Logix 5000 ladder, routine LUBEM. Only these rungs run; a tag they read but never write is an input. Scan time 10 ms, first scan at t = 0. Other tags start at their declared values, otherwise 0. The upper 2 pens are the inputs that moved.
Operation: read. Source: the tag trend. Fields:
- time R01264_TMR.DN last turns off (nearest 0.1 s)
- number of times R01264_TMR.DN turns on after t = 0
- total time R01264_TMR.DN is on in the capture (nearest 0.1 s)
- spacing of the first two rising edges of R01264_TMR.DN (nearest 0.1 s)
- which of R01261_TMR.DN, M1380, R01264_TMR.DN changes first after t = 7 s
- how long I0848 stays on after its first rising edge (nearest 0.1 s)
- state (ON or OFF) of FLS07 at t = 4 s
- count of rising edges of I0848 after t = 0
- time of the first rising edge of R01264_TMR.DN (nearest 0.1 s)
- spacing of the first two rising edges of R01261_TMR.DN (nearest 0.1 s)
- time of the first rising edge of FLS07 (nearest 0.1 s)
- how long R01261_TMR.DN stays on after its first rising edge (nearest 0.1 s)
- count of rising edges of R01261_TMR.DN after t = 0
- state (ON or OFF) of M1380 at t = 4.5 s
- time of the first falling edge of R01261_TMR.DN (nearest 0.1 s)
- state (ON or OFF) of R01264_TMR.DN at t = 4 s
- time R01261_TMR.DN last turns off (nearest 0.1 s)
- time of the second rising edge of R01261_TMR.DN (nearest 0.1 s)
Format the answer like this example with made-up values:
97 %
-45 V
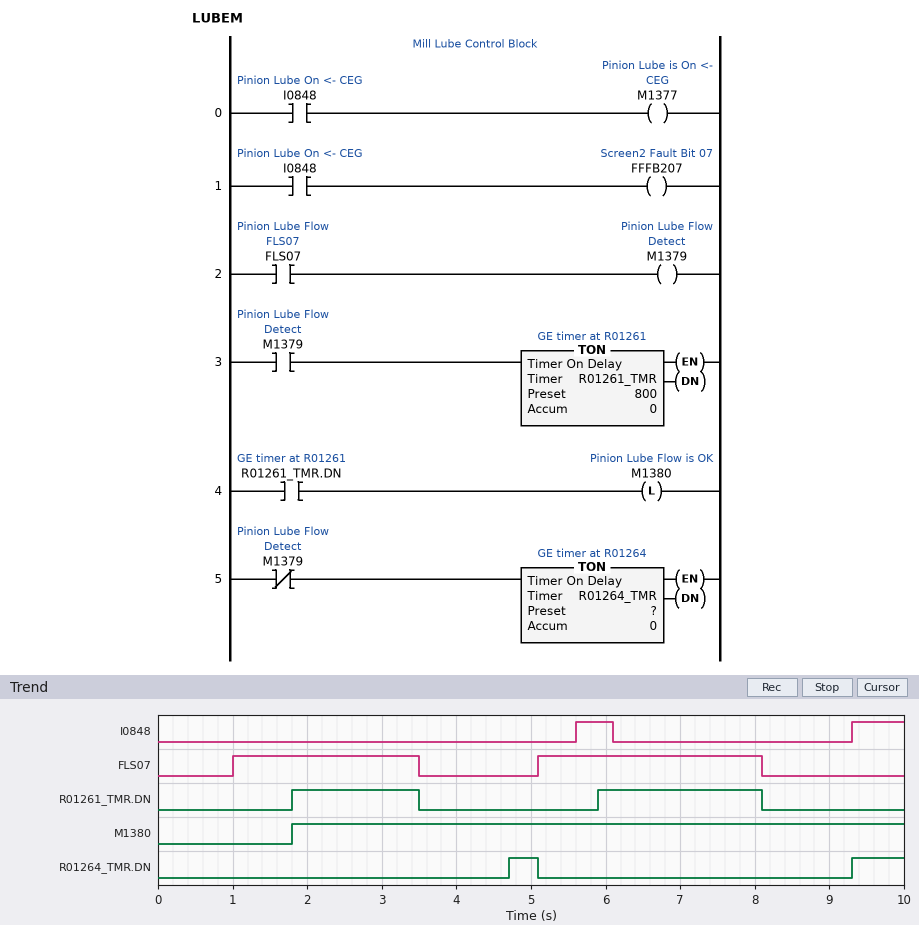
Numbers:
5.1 s
2
1.1 s
4.6 s
R01261_TMR.DN
0.5 s
OFF
2
4.7 s
4.1 s
1.0 s
1.7 s
2
ON
3.5 s
OFF
8.1 s
5.9 s
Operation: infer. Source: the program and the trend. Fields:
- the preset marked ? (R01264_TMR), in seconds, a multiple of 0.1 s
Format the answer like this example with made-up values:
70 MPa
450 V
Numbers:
1.2 s
